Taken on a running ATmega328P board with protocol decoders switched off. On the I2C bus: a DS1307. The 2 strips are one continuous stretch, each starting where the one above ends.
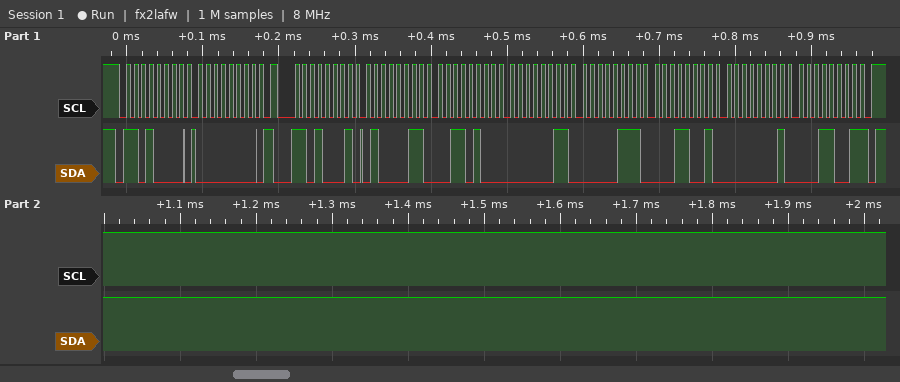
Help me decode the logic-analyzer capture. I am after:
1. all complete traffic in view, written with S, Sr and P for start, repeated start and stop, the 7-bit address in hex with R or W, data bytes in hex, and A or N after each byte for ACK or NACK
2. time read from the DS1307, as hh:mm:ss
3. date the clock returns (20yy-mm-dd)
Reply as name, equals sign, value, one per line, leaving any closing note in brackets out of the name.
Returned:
all complete traffic in view, written with S, Sr and P for start, repeated start and stop, the 7-bit address in hex with R or W, data bytes in hex, and A or N after each byte for ACK or NACK = S 68W A 00 A Sr 68R A 43 A 34 A 03 A 07 A 19 A 01 A 19 N P
time read from the DS1307, as hh:mm:ss = 03:34:43
date the clock returns = 2019-01-19
